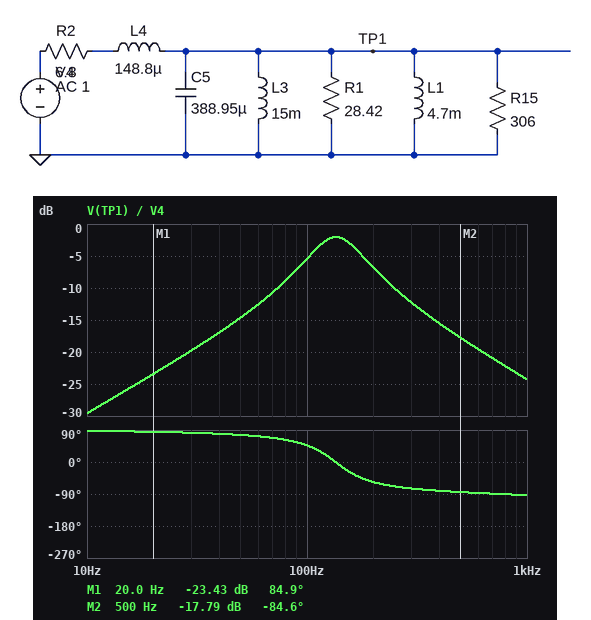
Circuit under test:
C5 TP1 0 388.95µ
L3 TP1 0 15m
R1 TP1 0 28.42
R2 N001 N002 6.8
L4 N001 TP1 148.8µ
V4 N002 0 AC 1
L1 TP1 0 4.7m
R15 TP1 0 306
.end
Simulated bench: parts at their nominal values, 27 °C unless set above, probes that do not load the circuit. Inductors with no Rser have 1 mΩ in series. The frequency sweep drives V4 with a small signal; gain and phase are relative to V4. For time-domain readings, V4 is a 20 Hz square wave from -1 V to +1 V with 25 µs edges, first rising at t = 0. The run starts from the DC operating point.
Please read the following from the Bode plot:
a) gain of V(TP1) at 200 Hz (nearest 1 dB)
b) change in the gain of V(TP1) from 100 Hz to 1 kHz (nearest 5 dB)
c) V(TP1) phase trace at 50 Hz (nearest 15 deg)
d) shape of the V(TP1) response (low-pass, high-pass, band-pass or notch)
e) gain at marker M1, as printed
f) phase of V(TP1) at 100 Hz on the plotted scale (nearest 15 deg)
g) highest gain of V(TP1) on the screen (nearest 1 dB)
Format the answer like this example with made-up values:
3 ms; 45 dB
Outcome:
-7 dB; -20 dB; 75 deg; band-pass; -23.43 dB; 45 deg; -2 dB
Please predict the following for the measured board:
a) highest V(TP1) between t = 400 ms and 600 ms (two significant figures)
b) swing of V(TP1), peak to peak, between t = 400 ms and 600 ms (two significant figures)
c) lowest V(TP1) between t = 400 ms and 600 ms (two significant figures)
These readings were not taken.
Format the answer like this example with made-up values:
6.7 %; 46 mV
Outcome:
610 mV; 1.2 V; -610 mV
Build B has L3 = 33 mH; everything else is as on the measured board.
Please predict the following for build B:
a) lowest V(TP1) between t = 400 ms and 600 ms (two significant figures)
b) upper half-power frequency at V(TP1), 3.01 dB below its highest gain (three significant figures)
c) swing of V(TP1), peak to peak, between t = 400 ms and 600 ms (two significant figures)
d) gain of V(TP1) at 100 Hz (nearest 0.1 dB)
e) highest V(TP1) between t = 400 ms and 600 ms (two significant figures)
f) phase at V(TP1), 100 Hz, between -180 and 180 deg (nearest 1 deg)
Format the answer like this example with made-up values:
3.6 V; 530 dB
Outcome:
-640 mV; 170 Hz; 1.3 V; -4.1 dB; 640 mV; 37 deg
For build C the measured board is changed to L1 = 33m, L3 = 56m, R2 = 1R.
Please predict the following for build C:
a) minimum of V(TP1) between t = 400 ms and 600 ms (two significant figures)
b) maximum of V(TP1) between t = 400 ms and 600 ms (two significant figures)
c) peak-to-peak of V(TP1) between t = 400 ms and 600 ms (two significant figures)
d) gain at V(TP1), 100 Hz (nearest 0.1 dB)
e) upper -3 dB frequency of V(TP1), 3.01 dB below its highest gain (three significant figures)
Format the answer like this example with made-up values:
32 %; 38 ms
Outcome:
-1.5 V; 1.5 V; 2.9 V; -0.3 dB; 586 Hz
